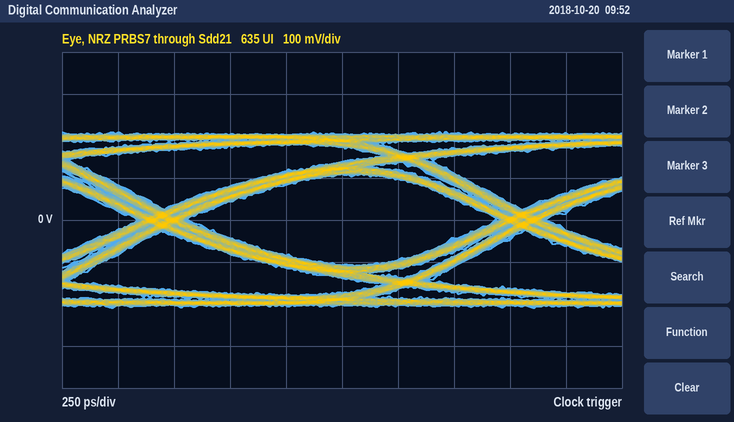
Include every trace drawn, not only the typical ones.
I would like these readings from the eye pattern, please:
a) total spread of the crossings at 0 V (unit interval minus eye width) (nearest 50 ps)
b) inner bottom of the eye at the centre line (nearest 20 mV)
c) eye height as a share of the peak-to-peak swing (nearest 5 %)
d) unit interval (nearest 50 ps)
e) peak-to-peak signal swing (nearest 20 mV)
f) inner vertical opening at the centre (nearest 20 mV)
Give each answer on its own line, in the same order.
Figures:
250 ps
-100 mV
50 %
1.60 ns
420 mV
220 mV
